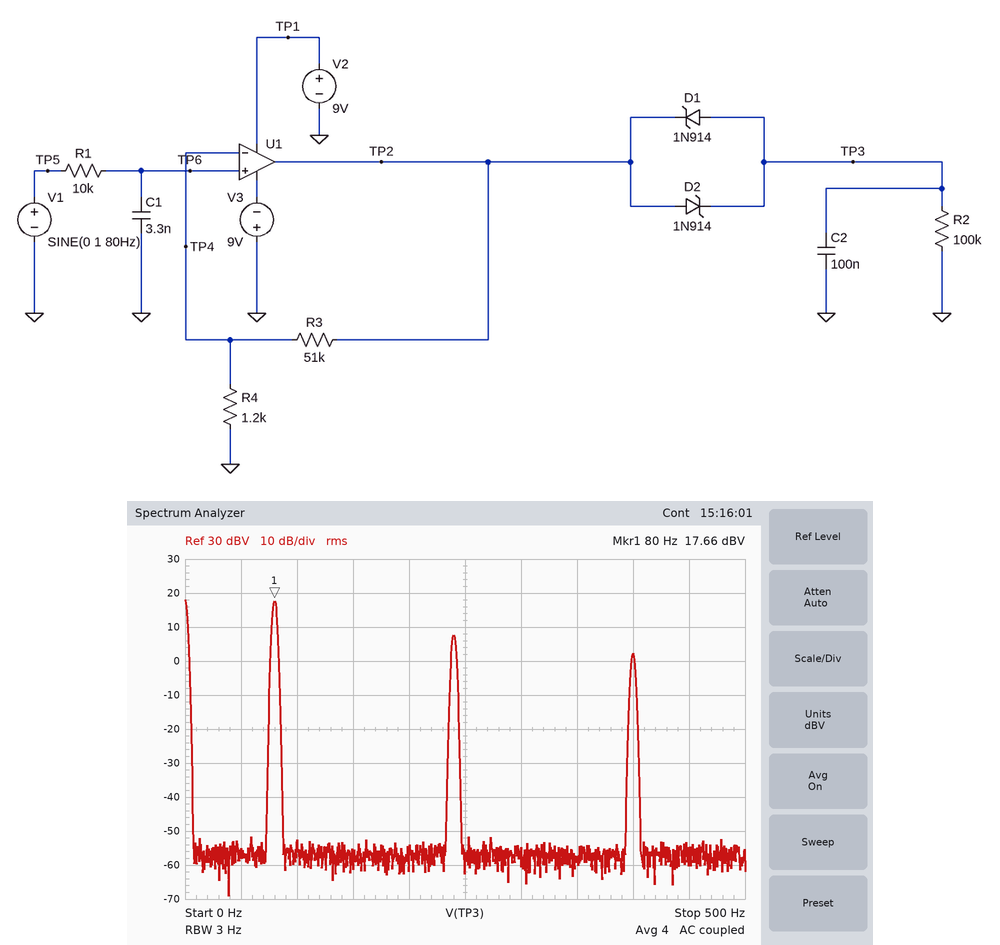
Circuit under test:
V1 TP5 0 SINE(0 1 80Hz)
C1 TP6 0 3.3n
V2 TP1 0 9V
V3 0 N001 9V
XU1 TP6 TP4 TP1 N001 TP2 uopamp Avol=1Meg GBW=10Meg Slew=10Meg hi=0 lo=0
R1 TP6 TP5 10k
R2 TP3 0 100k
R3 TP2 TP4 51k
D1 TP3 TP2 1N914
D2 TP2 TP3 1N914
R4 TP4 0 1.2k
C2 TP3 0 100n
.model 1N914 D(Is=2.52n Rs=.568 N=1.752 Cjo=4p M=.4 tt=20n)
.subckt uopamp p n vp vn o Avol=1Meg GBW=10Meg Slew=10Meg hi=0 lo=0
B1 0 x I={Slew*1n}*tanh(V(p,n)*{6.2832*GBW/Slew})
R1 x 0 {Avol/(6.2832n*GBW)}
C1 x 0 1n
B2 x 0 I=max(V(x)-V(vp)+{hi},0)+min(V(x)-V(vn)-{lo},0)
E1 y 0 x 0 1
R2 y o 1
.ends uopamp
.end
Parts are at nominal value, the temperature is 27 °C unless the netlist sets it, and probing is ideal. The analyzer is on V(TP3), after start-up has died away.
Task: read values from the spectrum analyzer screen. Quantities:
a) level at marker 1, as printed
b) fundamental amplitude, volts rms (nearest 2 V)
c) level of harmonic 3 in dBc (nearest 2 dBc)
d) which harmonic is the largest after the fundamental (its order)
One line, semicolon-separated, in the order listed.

17.66 dBV; 8 V; -10 dBc; 3
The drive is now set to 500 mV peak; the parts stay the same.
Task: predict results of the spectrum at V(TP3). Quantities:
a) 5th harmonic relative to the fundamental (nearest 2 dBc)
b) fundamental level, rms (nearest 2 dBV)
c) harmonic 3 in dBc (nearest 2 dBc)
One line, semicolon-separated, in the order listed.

-20 dBc; 18 dBV; -12 dBc
